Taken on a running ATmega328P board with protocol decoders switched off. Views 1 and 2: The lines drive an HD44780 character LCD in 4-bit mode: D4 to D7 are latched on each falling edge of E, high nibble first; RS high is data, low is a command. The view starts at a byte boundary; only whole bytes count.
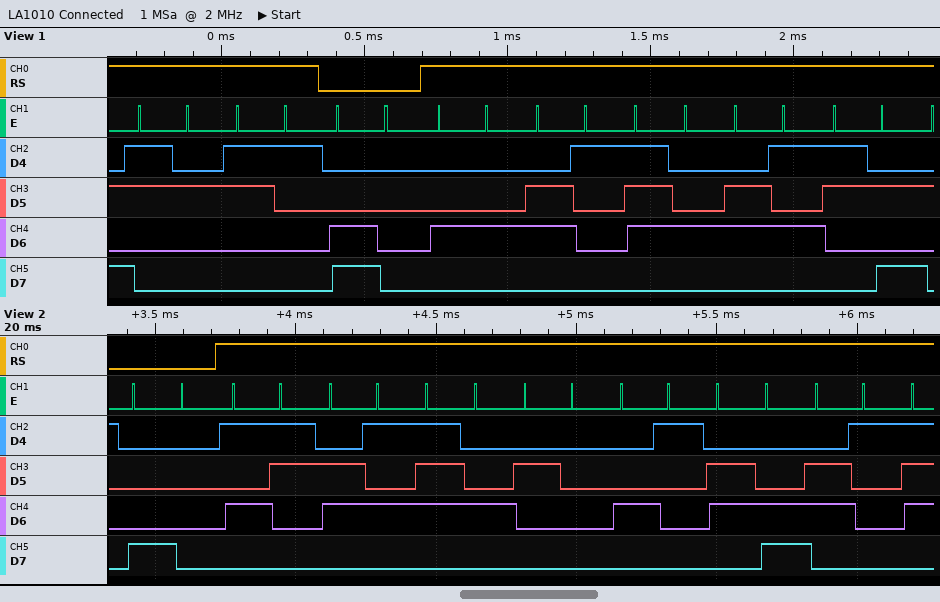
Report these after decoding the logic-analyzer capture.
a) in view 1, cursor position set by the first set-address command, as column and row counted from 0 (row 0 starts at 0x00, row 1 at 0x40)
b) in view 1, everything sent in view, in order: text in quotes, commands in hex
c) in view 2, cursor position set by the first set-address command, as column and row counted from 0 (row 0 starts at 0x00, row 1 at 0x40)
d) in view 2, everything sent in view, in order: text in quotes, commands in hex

column 0, row 1
"21" 0xC0 "Date:"
column 0, row 0
0x80 "Set Ala"
